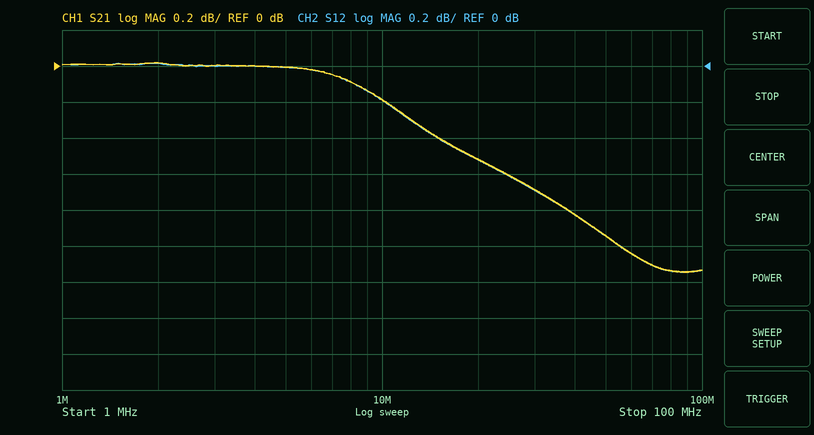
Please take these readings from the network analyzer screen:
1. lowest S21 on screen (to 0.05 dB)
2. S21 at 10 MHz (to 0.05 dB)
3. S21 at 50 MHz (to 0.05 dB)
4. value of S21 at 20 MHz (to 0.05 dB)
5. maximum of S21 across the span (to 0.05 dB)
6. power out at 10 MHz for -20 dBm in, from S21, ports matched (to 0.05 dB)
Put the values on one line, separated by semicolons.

-1.15 dB; -0.20 dB; -0.95 dB; -0.50 dB; 0.00 dB; -20.20 dBm
